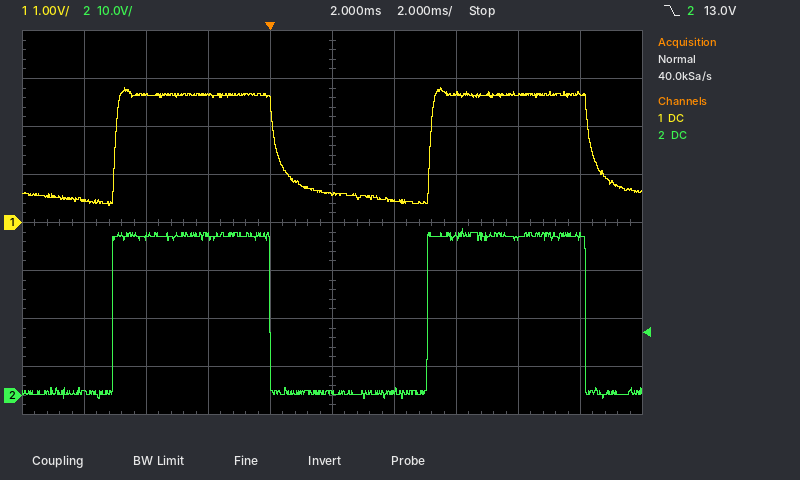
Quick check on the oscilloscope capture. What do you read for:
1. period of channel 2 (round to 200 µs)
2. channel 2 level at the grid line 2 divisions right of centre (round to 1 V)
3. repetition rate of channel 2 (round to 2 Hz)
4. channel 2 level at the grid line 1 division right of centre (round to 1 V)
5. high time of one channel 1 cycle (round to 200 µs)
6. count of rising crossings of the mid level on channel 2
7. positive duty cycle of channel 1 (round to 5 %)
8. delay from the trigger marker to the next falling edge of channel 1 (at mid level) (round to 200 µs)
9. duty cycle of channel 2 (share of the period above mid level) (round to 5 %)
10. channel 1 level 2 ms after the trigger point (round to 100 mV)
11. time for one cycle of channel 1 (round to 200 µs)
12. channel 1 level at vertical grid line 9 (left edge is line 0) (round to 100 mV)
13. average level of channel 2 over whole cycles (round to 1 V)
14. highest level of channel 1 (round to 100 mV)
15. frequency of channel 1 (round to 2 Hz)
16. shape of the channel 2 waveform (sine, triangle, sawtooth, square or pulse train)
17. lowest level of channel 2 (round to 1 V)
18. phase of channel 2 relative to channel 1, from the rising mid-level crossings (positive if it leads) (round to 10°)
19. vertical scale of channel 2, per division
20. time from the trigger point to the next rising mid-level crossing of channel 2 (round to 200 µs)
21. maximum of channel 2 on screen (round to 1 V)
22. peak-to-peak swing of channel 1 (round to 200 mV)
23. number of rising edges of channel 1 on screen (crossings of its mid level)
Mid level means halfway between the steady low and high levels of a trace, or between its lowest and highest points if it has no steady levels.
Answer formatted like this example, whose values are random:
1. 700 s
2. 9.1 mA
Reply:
1. 10.2 ms
2. 33 V
3. 98 Hz
4. 1 V
5. 5.2 ms
6. 2
7. 50 %
8. 200 µs
9. 50 %
10. 600 mV
11. 10.2 ms
12. 2.7 V
13. 17 V
14. 2.8 V
15. 98 Hz
16. square
17. -1 V
18. 0°
19. 10 V
20. 5.0 ms
21. 35 V
22. 2.4 V
23. 2
